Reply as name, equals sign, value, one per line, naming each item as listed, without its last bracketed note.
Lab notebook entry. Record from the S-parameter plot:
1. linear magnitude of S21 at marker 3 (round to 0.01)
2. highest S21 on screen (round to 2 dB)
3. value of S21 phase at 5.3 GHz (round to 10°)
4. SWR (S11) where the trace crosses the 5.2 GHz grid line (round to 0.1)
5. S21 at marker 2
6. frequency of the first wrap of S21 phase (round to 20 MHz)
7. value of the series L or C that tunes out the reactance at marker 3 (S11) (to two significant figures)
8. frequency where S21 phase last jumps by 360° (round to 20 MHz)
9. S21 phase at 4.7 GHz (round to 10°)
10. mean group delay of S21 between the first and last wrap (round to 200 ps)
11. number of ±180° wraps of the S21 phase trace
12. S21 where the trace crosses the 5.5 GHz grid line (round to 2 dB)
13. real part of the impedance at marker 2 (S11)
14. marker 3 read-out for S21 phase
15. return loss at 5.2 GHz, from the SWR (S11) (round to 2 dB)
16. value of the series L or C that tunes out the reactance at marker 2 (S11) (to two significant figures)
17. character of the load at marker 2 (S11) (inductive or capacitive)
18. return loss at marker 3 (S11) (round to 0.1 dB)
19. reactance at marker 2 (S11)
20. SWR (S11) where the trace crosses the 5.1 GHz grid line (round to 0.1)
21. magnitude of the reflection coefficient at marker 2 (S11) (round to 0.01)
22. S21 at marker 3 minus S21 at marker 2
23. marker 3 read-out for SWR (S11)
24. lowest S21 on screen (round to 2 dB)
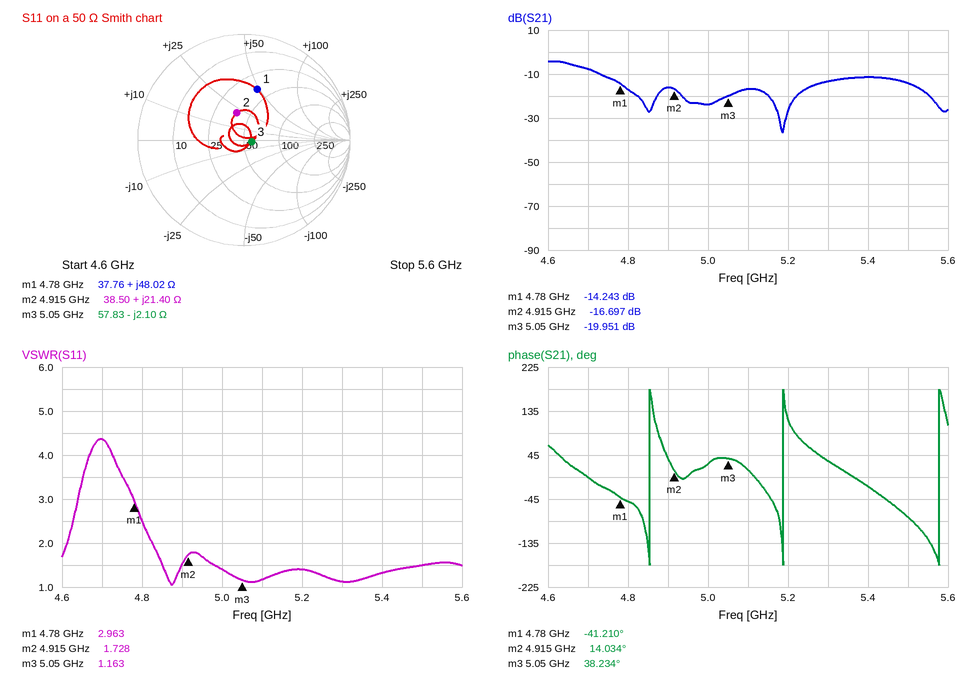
linear magnitude of S21 at marker 3 = 0.10
highest S21 on screen = -4 dB
value of S21 phase at 5.3 GHz = 30°
SWR (S11) where the trace crosses the 5.2 GHz grid line = 1.4
S21 at marker 2 = -16.697 dB
frequency of the first wrap of S21 phase = 4.86 GHz
value of the series L or C that tunes out the reactance at marker 3 (S11) = 66 pH
frequency where S21 phase last jumps by 360° = 5.58 GHz
S21 phase at 4.7 GHz = 0°
mean group delay of S21 between the first and last wrap = 2.8 ns
number of ±180° wraps of the S21 phase trace = 3
S21 where the trace crosses the 5.5 GHz grid line = -14 dB
real part of the impedance at marker 2 = 38.50 Ω
marker 3 read-out for S21 phase = 38.234°
return loss at 5.2 GHz, from the SWR (S11) = 16 dB
value of the series L or C that tunes out the reactance at marker 2 (S11) = 1.5 pF
character of the load at marker 2 (S11) = inductive
return loss at marker 3 (S11) = 22.5 dB
reactance at marker 2 = +21.40 Ω
SWR (S11) where the trace crosses the 5.1 GHz grid line = 1.2
magnitude of the reflection coefficient at marker 2 (S11) = 0.27
S21 at marker 3 minus S21 at marker 2 = -3.254 dB
marker 3 read-out for SWR = 1.163
lowest S21 on screen = -36 dB
